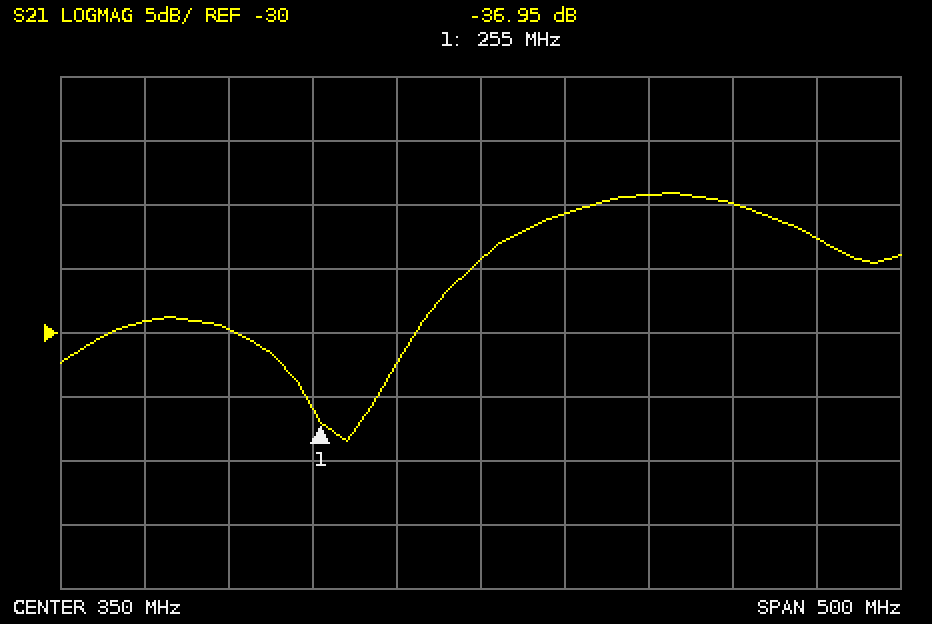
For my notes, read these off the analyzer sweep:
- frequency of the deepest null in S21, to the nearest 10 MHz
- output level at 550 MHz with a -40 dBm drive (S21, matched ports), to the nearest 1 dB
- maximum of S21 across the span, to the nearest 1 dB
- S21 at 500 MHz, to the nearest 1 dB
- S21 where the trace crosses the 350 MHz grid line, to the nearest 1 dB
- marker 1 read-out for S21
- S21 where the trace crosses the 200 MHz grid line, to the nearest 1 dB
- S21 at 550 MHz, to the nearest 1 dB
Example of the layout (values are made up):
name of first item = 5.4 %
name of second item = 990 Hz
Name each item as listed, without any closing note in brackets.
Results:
frequency of the deepest null in S21, to the nearest 10 MHz = 270 MHz
output level at 550 MHz with a -40 dBm drive (S21, matched ports), to the nearest 1 dB = -63 dBm
maximum of S21 across the span, to the nearest 1 dB = -19 dB
S21 at 500 MHz, to the nearest 1 dB = -20 dB
S21 where the trace crosses the 350 MHz grid line, to the nearest 1 dB = -24 dB
marker 1 read-out for S21 = -36.95 dB
S21 where the trace crosses the 200 MHz grid line, to the nearest 1 dB = -30 dB
S21 at 550 MHz, to the nearest 1 dB = -23 dB
